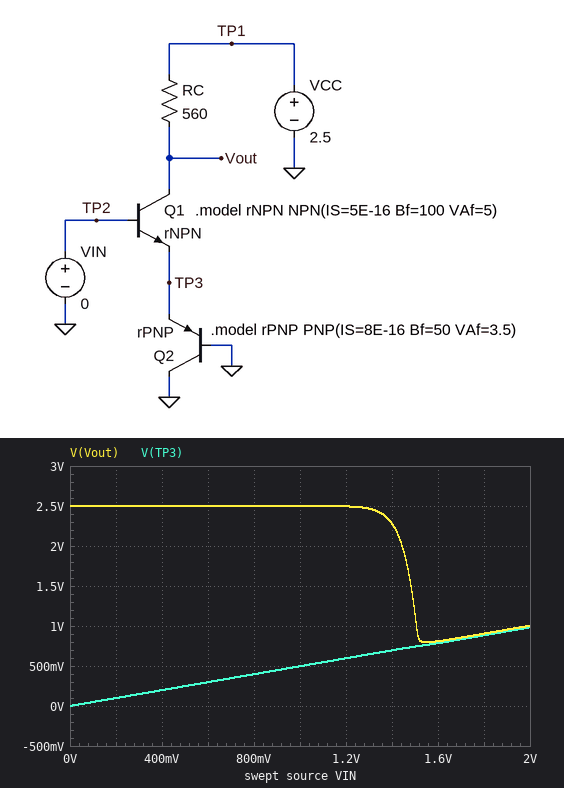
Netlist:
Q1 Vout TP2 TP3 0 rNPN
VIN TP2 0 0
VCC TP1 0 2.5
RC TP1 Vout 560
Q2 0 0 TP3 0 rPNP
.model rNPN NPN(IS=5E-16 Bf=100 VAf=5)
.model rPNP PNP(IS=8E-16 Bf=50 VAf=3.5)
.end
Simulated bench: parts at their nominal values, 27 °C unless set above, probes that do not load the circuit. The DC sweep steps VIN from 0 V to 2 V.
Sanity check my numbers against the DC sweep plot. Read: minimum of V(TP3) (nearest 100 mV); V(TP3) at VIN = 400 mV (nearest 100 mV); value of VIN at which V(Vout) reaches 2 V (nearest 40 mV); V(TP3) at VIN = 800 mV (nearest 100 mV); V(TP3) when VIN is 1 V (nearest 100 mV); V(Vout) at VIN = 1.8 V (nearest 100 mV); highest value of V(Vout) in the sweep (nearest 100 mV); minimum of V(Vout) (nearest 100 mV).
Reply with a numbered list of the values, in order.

1. 0 V
2. 200 mV
3. 1.44 V
4. 400 mV
5. 500 mV
6. 900 mV
7. 2.5 V
8. 800 mV
